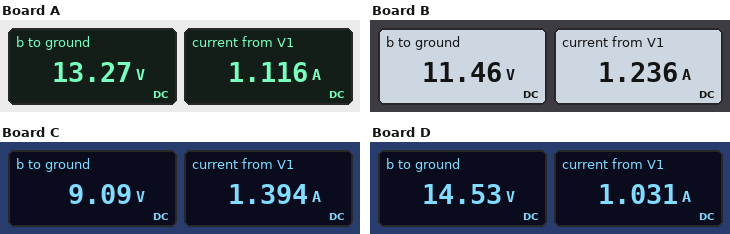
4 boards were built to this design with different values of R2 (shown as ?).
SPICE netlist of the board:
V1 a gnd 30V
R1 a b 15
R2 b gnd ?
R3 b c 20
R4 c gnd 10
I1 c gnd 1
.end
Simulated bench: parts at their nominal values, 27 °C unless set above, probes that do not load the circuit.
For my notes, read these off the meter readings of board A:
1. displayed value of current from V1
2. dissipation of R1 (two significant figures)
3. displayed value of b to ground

1.116 A
19 W
13.27 V
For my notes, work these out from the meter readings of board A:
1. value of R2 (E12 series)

39 Ω
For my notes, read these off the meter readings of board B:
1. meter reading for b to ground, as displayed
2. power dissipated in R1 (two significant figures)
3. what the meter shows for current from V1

11.46 V
23 W
1.236 A
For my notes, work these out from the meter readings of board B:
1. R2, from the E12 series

22 Ω
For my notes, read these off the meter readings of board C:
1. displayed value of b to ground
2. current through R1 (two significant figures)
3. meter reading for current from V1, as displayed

9.09 V
1.4 A
1.394 A
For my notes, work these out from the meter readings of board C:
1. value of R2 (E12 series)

12 Ω
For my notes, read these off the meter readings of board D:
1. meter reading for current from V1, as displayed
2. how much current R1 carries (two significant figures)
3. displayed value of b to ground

1.031 A
1.0 A
14.53 V
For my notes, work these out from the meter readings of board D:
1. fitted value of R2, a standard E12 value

68 Ω
